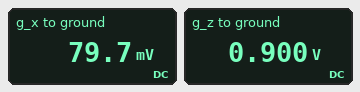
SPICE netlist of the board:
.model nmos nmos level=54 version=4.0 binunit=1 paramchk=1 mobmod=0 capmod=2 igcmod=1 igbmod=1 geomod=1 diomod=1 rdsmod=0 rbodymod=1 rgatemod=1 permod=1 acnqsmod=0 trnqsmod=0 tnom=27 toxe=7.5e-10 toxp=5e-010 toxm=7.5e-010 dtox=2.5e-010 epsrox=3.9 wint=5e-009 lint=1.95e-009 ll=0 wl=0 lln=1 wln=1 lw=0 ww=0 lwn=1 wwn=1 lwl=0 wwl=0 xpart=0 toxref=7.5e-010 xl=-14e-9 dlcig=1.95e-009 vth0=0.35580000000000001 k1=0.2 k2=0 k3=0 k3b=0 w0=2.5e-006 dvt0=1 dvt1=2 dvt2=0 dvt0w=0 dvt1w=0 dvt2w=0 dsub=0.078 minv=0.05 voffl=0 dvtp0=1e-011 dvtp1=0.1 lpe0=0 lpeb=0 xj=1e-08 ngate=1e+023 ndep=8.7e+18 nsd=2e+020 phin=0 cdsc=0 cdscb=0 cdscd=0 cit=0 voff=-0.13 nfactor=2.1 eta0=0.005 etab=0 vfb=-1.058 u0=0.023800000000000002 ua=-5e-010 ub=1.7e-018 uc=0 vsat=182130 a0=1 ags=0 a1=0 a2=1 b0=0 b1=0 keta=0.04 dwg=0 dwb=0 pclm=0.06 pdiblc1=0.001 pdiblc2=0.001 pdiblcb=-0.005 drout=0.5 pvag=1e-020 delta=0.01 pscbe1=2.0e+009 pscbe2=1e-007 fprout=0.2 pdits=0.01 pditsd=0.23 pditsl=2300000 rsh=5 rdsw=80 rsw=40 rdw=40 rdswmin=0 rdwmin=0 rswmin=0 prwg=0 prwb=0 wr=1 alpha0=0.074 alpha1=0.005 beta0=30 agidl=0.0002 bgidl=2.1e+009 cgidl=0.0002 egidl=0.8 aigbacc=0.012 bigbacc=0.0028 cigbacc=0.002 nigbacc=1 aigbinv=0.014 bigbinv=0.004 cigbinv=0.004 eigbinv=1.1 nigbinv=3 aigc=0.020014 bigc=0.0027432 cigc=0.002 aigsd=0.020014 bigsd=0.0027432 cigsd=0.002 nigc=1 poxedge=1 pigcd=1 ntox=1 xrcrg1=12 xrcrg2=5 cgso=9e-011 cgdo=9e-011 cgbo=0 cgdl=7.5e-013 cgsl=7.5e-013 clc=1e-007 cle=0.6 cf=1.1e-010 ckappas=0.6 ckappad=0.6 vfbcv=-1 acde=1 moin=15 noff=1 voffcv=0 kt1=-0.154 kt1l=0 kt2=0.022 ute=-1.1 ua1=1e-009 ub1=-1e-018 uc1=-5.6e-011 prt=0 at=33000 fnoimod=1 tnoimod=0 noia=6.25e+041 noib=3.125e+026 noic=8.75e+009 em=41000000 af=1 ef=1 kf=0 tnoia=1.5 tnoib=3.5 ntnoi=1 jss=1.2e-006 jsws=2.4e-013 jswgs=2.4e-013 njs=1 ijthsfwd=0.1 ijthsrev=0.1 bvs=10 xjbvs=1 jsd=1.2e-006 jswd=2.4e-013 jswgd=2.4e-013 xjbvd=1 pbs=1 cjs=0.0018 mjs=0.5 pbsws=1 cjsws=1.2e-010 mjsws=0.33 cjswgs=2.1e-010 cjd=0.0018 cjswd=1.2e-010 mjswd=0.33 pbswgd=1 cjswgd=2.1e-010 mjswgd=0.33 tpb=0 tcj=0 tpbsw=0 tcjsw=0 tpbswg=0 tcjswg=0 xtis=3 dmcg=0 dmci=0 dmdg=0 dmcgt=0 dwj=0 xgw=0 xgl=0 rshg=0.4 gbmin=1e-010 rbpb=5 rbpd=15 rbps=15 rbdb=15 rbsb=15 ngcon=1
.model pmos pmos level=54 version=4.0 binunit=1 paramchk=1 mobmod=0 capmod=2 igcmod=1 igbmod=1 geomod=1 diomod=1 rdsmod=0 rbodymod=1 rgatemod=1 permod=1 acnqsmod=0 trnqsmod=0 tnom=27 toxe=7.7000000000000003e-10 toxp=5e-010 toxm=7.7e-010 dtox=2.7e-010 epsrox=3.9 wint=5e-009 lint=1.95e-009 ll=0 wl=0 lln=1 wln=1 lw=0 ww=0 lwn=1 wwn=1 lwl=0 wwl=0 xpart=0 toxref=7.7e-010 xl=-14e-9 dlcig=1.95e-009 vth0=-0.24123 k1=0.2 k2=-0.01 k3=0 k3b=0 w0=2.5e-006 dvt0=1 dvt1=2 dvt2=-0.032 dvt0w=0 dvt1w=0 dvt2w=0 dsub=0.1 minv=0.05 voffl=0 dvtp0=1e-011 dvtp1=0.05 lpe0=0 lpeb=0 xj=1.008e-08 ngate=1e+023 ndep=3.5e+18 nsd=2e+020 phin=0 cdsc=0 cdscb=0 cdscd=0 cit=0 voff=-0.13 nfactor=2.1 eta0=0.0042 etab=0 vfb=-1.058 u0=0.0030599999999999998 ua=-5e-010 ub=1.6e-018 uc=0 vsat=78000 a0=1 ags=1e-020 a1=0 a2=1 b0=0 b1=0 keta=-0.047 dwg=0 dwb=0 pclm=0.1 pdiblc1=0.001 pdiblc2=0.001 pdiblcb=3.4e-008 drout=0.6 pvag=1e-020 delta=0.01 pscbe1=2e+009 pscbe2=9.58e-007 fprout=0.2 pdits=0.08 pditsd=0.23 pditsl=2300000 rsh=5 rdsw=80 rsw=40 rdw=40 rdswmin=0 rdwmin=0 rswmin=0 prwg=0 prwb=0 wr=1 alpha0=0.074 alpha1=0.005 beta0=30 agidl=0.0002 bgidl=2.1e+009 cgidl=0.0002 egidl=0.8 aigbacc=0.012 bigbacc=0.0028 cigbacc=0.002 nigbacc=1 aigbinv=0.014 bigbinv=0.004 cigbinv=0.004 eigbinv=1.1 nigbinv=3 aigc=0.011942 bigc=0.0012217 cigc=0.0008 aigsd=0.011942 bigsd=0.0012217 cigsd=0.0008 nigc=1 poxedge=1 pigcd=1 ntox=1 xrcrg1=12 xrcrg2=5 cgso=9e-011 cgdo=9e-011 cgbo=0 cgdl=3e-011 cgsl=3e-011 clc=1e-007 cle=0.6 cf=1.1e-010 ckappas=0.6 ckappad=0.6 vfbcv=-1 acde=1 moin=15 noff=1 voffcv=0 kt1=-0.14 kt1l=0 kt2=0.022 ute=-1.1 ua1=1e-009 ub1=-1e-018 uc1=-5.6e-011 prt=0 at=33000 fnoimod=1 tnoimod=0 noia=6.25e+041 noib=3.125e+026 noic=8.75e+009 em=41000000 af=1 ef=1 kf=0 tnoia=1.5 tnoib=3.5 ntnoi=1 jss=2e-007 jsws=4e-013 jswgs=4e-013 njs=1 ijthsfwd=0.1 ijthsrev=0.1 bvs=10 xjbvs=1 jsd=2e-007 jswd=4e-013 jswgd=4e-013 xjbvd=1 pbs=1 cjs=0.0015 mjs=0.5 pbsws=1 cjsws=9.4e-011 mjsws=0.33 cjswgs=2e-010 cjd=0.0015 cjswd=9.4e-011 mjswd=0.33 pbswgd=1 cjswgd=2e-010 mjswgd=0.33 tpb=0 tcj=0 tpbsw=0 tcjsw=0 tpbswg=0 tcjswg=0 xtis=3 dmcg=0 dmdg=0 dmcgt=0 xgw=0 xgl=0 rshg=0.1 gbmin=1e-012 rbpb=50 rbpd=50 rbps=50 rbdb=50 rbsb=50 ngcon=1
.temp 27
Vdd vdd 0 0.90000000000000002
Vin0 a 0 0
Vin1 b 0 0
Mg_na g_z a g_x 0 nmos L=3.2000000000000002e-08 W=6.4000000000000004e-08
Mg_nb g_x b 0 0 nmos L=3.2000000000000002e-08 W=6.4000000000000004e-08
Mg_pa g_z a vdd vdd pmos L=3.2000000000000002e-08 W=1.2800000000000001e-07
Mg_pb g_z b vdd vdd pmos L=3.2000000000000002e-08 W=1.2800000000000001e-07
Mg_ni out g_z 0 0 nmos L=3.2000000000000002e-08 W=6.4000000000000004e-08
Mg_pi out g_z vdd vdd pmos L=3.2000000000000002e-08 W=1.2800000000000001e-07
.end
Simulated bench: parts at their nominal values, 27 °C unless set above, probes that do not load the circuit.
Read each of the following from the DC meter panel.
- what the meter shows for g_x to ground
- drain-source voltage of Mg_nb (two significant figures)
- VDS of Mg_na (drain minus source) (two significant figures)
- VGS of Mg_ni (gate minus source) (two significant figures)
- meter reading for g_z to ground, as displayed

79.7 mV
80 mV
820 mV
900 mV
0.900 V
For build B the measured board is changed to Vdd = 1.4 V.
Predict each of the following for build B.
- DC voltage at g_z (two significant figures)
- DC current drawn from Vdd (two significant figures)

1.4 V
4.8 µA
